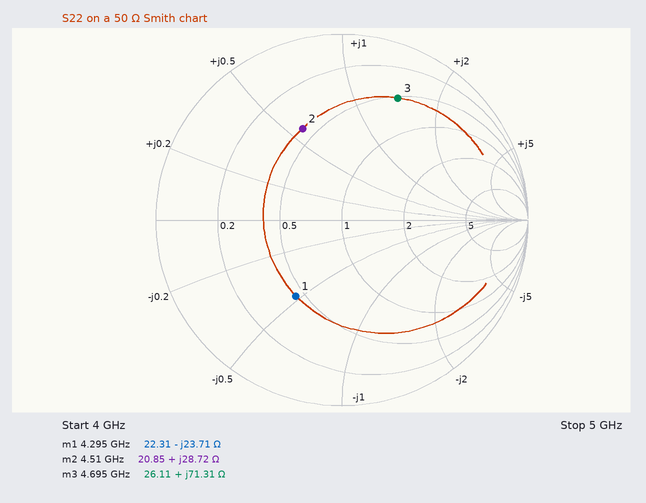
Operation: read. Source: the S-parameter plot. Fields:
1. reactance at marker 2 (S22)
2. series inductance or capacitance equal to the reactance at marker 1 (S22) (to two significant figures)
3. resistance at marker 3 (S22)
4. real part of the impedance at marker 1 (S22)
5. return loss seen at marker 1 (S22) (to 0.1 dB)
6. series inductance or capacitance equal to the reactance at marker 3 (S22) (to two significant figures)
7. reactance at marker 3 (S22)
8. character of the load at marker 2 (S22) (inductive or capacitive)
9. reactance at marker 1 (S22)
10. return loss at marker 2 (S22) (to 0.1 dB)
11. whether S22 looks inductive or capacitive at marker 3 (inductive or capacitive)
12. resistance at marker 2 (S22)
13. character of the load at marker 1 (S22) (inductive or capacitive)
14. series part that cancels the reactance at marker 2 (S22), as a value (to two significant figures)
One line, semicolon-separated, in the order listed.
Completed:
+28.72 Ω; 1.6 pF; 26.11 Ω; 22.31 Ω; 6.4 dB; 2.4 nH; +71.31 Ω; inductive; -23.71 Ω; 5.4 dB; inductive; 20.85 Ω; capacitive; 1.2 pF
